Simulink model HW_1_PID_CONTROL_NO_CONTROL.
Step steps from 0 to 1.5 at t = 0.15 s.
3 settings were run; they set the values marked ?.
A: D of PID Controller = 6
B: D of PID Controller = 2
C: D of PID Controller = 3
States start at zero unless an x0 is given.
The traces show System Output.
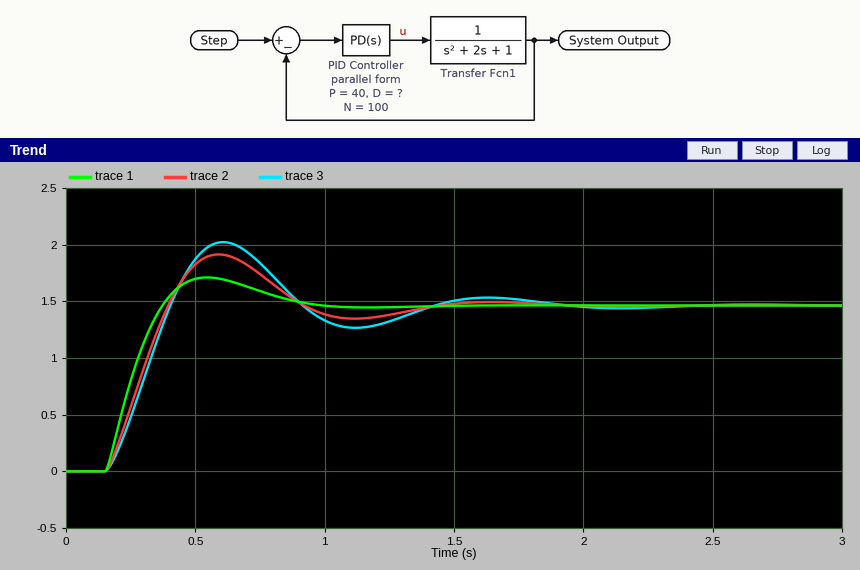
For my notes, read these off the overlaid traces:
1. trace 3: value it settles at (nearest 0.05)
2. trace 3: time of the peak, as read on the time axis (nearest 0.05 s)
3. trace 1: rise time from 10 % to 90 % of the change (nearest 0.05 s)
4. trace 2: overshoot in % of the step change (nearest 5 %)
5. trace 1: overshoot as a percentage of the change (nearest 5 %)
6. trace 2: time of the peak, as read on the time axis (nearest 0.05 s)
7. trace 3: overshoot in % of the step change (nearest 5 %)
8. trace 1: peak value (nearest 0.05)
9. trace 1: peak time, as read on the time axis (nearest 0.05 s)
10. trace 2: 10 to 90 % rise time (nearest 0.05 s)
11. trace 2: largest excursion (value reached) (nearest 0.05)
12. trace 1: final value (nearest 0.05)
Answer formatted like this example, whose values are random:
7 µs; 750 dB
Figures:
1.45; 0.60 s; 0.15 s; 30 %; 15 %; 0.60 s; 40 %; 1.70; 0.55 s; 0.20 s; 1.90; 1.45
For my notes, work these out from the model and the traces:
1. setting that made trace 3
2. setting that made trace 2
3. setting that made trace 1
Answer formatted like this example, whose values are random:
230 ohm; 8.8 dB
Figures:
B; C; A
